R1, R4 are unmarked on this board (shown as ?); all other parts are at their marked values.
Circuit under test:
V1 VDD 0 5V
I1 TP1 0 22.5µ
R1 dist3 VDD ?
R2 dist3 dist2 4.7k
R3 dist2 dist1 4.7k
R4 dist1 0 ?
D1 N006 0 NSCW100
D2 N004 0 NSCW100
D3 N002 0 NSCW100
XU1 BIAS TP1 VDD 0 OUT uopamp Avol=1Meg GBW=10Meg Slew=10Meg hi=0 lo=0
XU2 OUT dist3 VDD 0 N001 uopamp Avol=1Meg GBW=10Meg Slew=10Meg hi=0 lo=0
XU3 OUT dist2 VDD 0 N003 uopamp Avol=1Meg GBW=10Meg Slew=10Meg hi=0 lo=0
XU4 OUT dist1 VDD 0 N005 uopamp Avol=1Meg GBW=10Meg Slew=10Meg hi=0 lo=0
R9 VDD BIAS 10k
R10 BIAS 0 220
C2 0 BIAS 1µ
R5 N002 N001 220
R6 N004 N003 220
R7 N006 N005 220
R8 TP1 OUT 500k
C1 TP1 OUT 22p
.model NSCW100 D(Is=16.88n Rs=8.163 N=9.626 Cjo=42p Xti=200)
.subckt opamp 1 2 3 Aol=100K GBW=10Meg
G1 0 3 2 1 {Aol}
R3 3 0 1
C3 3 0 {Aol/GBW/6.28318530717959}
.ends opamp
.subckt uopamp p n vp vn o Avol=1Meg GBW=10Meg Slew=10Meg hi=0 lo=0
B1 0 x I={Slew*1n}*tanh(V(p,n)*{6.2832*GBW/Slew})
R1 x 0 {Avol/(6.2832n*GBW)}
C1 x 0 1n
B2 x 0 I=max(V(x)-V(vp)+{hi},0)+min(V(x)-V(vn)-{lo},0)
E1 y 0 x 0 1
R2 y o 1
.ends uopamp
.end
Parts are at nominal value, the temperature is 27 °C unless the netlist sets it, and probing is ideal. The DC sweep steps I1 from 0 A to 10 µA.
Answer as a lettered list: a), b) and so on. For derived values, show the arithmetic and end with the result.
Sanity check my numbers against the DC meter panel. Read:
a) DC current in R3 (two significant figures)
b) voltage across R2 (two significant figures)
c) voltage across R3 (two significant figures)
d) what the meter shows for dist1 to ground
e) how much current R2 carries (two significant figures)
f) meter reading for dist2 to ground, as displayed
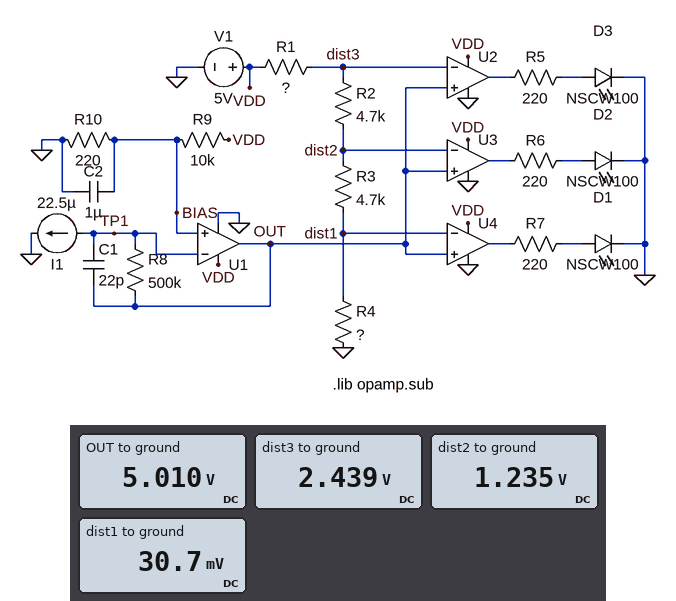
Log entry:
a) (1.235 V - 30.7 mV) / 4.7 kΩ = 260 µA
b) 2.439 V - 1.235 V = 1.2 V
c) 1.235 V - 30.7 mV = 1.2 V
d) 30.7 mV
e) (2.439 V - 1.235 V) / 4.7 kΩ = 260 µA
f) 1.235 V
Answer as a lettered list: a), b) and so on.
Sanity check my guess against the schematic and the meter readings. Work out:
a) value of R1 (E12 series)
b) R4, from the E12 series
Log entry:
a) 10 kΩ
b) 120 Ω
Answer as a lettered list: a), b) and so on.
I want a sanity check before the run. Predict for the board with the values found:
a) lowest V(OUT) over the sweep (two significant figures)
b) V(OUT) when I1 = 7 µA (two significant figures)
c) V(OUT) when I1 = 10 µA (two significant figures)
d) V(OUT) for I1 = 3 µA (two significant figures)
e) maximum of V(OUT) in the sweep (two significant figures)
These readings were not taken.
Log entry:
a) 110 mV
b) 3.6 V
c) 5.0 V
d) 1.6 V
e) 5.0 V
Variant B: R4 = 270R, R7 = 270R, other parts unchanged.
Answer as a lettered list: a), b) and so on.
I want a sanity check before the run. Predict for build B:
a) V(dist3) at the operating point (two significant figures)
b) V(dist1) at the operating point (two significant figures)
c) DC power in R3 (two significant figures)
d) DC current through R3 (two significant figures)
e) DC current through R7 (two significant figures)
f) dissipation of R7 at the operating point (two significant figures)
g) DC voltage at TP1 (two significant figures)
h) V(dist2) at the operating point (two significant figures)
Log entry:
a) 2.5 V
b) 69 mV
c) 300 µW
d) 250 µA
e) 6.5 mA
f) 11 mW
g) -6.2 V
h) 1.3 V
